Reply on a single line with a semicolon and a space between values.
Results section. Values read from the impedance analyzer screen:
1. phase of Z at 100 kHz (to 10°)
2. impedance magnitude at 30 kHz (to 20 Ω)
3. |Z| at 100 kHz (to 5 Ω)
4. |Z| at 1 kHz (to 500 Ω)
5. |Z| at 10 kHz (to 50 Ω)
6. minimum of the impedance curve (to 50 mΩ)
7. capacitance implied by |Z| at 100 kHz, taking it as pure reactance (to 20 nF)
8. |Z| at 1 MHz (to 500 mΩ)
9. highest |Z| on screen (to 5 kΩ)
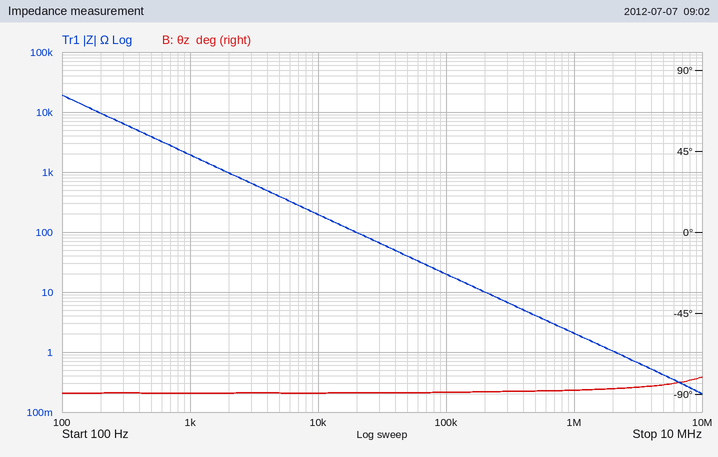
-90°; 60 Ω; 20 Ω; 2.0 kΩ; 200 Ω; 200 mΩ; 80 nF; 2.0 Ω; 20 kΩ
